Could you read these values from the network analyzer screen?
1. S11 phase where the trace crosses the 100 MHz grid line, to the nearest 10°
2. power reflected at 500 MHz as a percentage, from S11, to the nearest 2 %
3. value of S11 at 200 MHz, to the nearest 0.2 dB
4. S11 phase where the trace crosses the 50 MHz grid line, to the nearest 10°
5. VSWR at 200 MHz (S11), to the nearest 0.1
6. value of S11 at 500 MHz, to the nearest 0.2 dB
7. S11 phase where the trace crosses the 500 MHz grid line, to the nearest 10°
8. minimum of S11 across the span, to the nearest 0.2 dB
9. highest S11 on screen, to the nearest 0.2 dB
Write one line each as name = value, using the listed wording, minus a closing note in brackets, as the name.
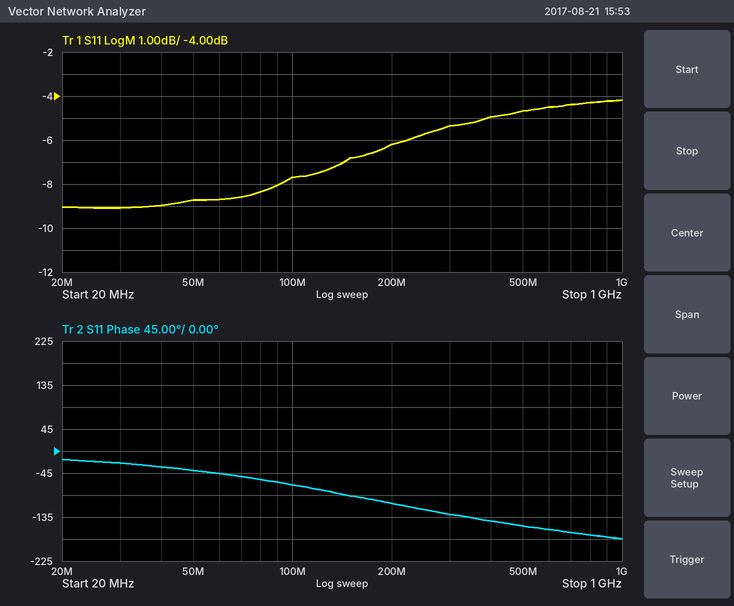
S11 phase where the trace crosses the 100 MHz grid line, to the nearest 10° = -70°
power reflected at 500 MHz as a percentage, from S11, to the nearest 2 % = 34 %
value of S11 at 200 MHz, to the nearest 0.2 dB = -6.2 dB
S11 phase where the trace crosses the 50 MHz grid line, to the nearest 10° = -40°
VSWR at 200 MHz (S11), to the nearest 0.1 = 2.9
value of S11 at 500 MHz, to the nearest 0.2 dB = -4.6 dB
S11 phase where the trace crosses the 500 MHz grid line, to the nearest 10° = -150°
minimum of S11 across the span, to the nearest 0.2 dB = -9.0 dB
highest S11 on screen, to the nearest 0.2 dB = -4.2 dB
